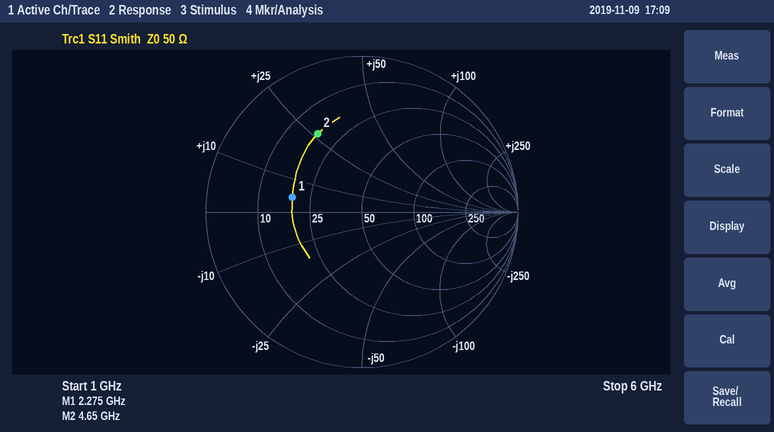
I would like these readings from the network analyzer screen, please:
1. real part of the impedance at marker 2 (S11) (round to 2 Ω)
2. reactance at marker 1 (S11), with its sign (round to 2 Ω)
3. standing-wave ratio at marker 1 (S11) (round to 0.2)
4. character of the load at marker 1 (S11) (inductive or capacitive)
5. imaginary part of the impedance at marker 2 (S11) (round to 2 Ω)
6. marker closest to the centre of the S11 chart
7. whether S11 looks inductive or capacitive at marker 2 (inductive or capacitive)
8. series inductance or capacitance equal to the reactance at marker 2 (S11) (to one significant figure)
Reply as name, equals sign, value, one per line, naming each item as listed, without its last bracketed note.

real part of the impedance at marker 2 (S11) = 18 Ω
reactance at marker 1 (S11), with its sign = +4 Ω
standing-wave ratio at marker 1 (S11) = 2.6
character of the load at marker 1 (S11) = inductive
imaginary part of the impedance at marker 2 (S11) = +26 Ω
marker closest to the centre of the S11 chart = marker 1
whether S11 looks inductive or capacitive at marker 2 = inductive
series inductance or capacitance equal to the reactance at marker 2 (S11) = 900 pH
